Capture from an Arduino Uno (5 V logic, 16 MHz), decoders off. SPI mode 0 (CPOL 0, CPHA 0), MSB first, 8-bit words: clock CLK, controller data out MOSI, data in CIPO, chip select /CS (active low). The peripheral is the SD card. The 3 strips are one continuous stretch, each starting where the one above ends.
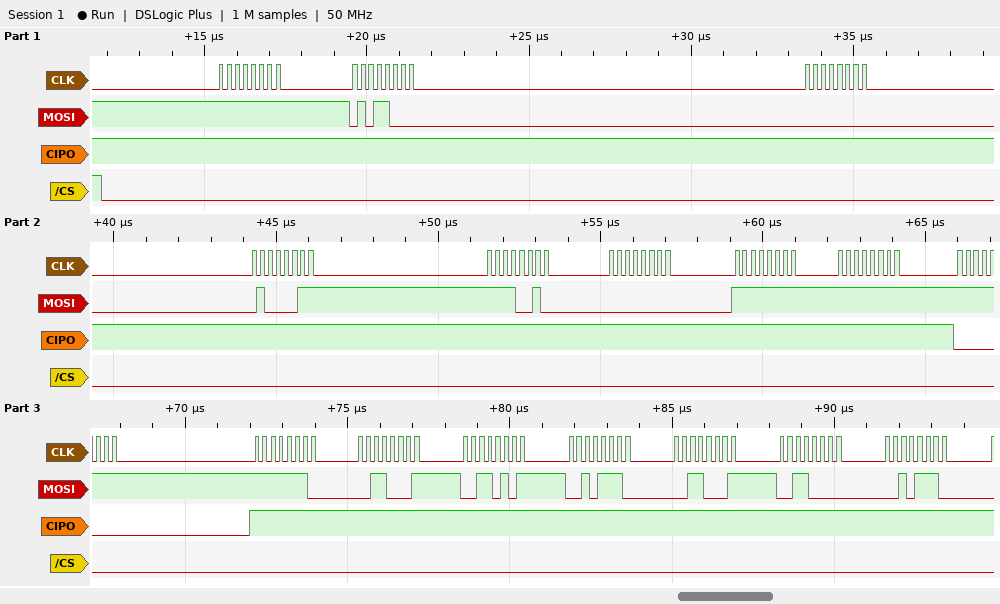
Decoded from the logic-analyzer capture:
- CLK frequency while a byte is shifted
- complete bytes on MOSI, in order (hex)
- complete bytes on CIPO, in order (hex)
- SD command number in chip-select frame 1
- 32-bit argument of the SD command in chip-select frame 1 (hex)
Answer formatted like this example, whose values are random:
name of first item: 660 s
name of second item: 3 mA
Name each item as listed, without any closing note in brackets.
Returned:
CLK frequency while a byte is shifted: 4 MHz
complete bytes on MOSI, in order: FF 58 00 43 F2 00 FF FF FF FE 31 35 2E 31 30 2E
complete bytes on CIPO, in order: FF FF FF FF FF FF FF FF 00 FF FF FF FF FF FF FF
SD command number in chip-select frame 1: CMD24
32-bit argument of the SD command in chip-select frame 1: 0x0043F200
